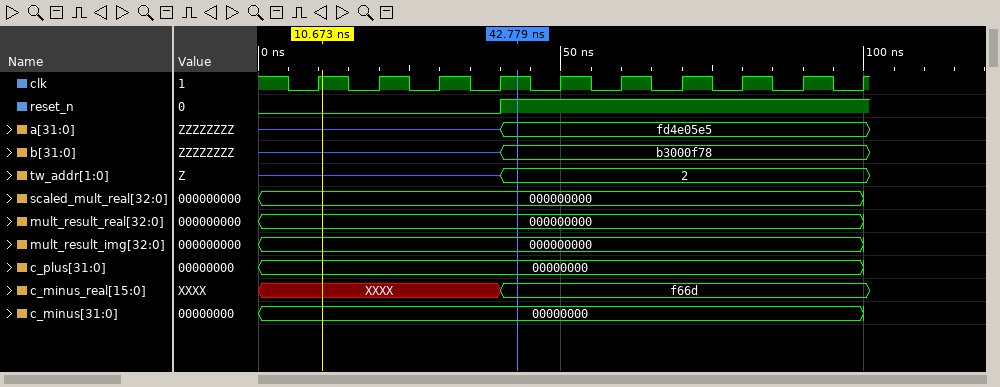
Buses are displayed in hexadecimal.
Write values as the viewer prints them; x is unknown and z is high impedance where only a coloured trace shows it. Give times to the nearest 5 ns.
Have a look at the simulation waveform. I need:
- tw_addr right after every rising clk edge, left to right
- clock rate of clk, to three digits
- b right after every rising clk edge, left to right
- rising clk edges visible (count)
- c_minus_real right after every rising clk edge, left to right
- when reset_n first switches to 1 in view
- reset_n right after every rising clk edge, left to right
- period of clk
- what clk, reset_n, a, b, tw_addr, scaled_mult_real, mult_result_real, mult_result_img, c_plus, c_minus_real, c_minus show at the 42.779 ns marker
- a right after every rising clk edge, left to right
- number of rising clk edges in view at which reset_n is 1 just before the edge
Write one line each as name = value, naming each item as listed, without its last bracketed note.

tw_addr right after every rising clk edge, left to right = z, z, z, 2, 2, 2, 2, 2, 2, 2
clock rate of clk, to three digits = 100 MHz
b right after every rising clk edge, left to right = z, z, z, b3000f78, b3000f78, b3000f78, b3000f78, b3000f78, b3000f78, b3000f78
rising clk edges visible = 10
c_minus_real right after every rising clk edge, left to right = XXXX, XXXX, XXXX, f66d, f66d, f66d, f66d, f66d, f66d, f66d
when reset_n first switches to 1 in view = 40 ns
reset_n right after every rising clk edge, left to right = 0 0 0 1 1 1 1 1 1 1
period of clk = 10 ns
what clk, reset_n, a, b, tw_addr, scaled_mult_real, mult_result_real, mult_result_img, c_plus, c_minus_real, c_minus show at the 42.779 ns marker = clk=1, reset_n=1, a=fd4e05e5, b=b3000f78, tw_addr=2, scaled_mult_real=000000000, mult_result_real=000000000, mult_result_img=000000000, c_plus=00000000, c_minus_real=f66d, c_minus=00000000
a right after every rising clk edge, left to right = z, z, z, fd4e05e5, fd4e05e5, fd4e05e5, fd4e05e5, fd4e05e5, fd4e05e5, fd4e05e5
number of rising clk edges in view at which reset_n is 1 just before the edge = 6
